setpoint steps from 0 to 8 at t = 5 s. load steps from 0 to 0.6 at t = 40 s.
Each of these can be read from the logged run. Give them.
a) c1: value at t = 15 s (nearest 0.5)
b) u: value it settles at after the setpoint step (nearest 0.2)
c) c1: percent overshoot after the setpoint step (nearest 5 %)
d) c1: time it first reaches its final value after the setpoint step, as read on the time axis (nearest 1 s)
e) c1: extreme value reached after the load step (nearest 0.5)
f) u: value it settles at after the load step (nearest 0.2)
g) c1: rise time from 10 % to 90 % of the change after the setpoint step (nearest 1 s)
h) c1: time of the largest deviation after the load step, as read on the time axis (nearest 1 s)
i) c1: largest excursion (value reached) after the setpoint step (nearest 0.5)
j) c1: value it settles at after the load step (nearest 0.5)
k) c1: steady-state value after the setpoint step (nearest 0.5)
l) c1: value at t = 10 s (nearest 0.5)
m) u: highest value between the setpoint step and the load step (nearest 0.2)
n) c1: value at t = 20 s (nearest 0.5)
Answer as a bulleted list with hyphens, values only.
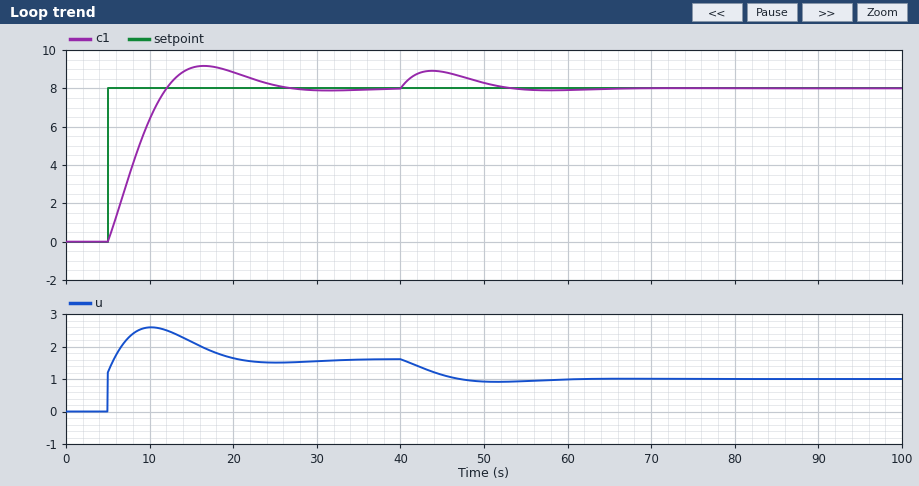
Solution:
- 9.0
- 1.6
- 15 %
- 12 s
- 9.0
- 1.0
- 5 s
- 44 s
- 9.0
- 8.0
- 8.0
- 6.5
- 2.6
- 9.0
